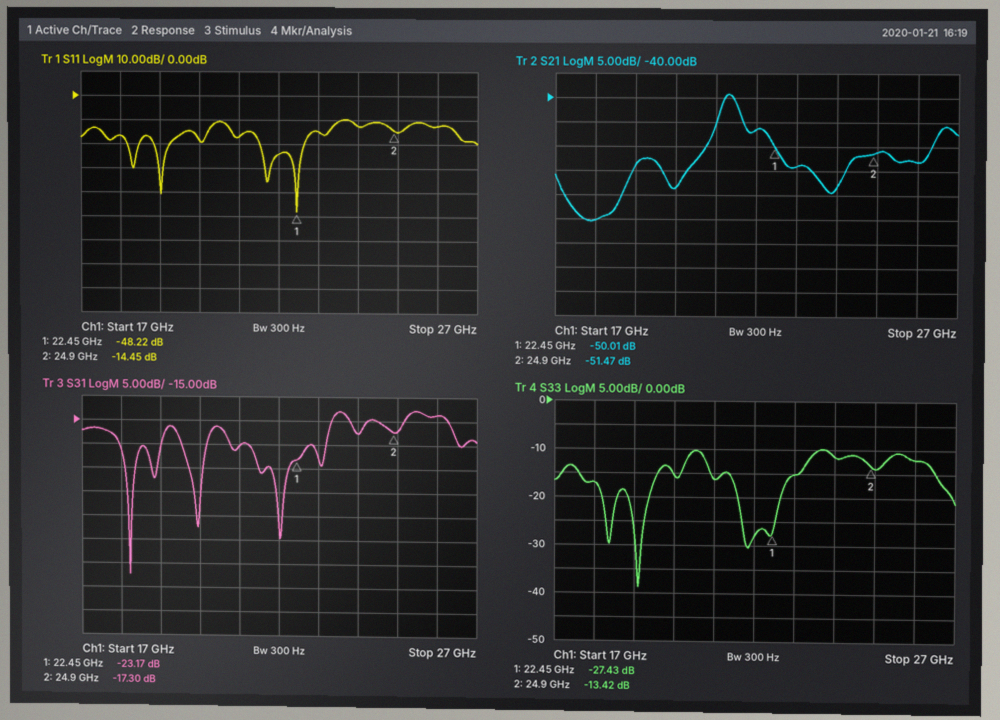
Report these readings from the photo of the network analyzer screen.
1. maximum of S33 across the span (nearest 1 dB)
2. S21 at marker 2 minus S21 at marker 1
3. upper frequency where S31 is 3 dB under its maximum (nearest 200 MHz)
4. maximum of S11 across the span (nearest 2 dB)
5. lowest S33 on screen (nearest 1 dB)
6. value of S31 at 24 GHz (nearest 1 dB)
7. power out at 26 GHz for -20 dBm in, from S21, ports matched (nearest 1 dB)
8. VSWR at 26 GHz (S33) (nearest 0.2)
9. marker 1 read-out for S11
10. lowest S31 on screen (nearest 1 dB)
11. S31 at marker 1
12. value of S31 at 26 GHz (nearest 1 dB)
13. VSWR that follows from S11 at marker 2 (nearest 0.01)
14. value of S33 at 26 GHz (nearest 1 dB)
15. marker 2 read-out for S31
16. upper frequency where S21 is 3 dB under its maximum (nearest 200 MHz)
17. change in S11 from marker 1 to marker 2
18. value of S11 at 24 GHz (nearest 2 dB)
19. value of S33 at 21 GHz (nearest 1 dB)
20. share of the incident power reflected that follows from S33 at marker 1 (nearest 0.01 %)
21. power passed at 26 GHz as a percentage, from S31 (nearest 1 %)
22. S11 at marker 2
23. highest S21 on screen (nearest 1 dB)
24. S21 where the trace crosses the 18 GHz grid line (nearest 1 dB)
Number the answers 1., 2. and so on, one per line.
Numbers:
1. -10 dB
2. -1.46 dB
3. 26.4 GHz
4. -10 dB
5. -39 dB
6. -18 dB
7. -73 dBm
8. 1.6
9. -48.22 dB
10. -47 dB
11. -23.17 dB
12. -14 dB
13. 1.47
14. -12 dB
15. -17.30 dB
16. 21.6 GHz
17. 33.77 dB
18. -12 dB
19. -16 dB
20. 0.18 %
21. 4 %
22. -14.45 dB
23. -39 dB
24. -65 dB
